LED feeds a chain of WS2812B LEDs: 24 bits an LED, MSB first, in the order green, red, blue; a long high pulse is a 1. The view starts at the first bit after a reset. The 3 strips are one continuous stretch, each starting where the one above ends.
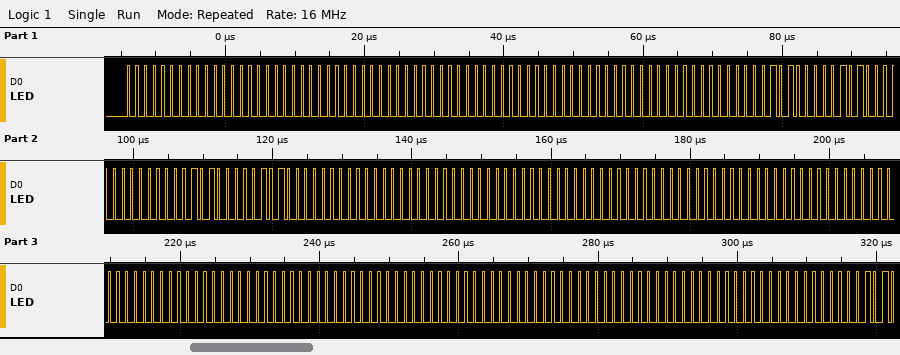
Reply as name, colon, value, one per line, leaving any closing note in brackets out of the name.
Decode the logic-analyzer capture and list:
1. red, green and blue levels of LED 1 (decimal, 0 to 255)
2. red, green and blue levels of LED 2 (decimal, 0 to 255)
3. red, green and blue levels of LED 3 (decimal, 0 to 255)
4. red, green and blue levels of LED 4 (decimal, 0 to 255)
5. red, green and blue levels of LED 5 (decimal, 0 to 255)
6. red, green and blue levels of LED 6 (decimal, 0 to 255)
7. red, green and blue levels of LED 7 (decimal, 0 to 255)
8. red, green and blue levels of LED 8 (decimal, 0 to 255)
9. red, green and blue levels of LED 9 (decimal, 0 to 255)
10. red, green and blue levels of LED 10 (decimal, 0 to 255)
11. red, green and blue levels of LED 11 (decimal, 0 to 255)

red, green and blue levels of LED 1: 0, 0, 0
red, green and blue levels of LED 2: 0, 0, 0
red, green and blue levels of LED 3: 0, 0, 0
red, green and blue levels of LED 4: 40, 40, 0
red, green and blue levels of LED 5: 40, 40, 0
red, green and blue levels of LED 6: 0, 0, 0
red, green and blue levels of LED 7: 0, 0, 0
red, green and blue levels of LED 8: 0, 0, 0
red, green and blue levels of LED 9: 0, 0, 0
red, green and blue levels of LED 10: 0, 0, 0
red, green and blue levels of LED 11: 0, 0, 0
